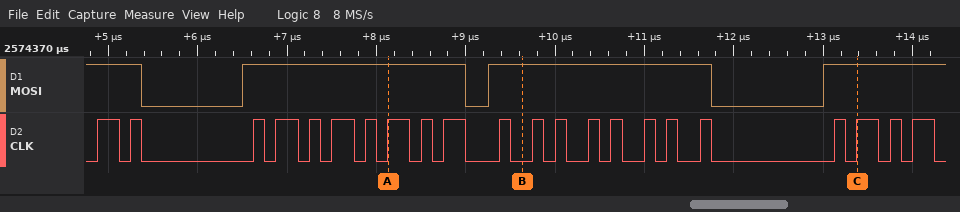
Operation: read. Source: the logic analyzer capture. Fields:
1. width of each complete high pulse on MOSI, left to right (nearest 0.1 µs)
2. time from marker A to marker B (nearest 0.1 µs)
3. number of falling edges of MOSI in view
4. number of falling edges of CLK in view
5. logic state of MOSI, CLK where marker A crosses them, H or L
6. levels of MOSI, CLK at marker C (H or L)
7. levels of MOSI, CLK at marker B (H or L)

2.5 µs, 2.5 µs
1.5 µs
3
22
MOSI=H, CLK=H
MOSI=H, CLK=H
MOSI=H, CLK=L
